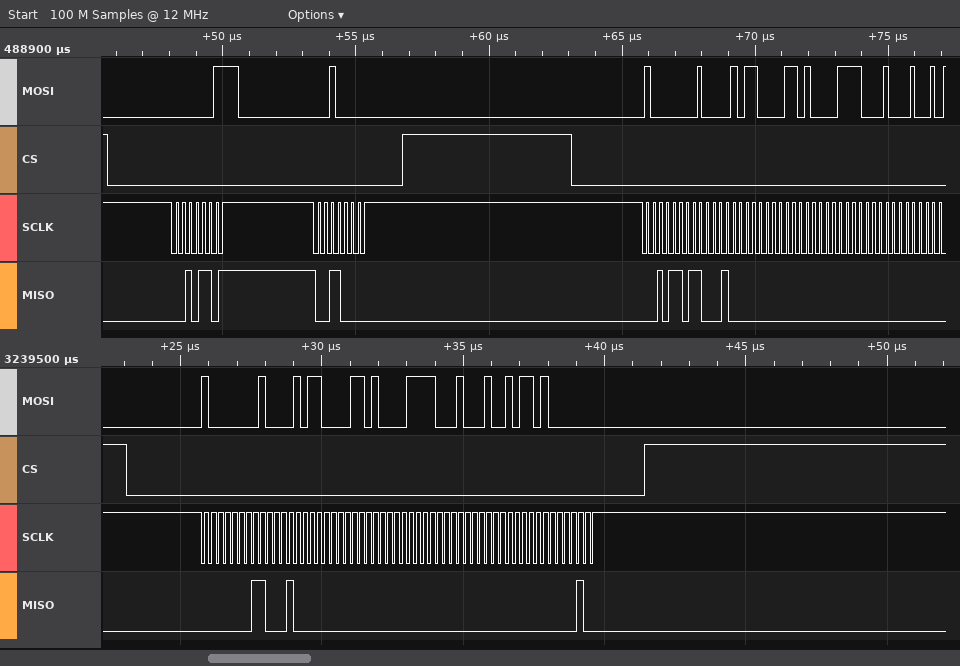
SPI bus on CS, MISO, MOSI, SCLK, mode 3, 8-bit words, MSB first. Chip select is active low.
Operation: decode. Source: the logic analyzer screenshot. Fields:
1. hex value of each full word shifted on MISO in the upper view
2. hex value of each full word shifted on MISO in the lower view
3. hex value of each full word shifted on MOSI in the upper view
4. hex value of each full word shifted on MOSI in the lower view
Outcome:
2D, 30, 2D, 88, 00, 00, 00
01, 88, 00, 00, 00, 00, 04
03, 20, 80, 85, 86, 87, 88
80, 85, 86, 87, 88, 96, 80
